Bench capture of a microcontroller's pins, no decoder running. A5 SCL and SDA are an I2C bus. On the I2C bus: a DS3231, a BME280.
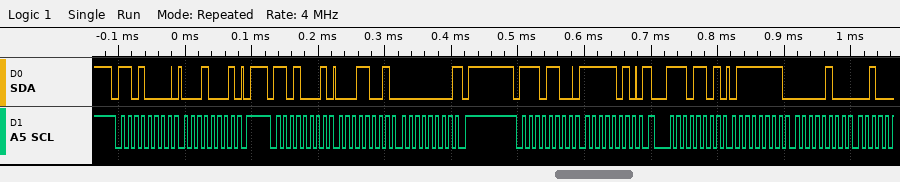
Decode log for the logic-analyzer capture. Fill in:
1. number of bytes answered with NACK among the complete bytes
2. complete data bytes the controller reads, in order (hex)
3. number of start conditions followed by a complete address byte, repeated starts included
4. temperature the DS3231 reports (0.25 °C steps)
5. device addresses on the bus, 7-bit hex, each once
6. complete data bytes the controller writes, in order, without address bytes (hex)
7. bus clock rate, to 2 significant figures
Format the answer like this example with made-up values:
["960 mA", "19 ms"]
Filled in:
["1", "19 00 7F 04", "4", "25.00 °C", "0x68 0x76", "11 FA", "100 kHz"]
